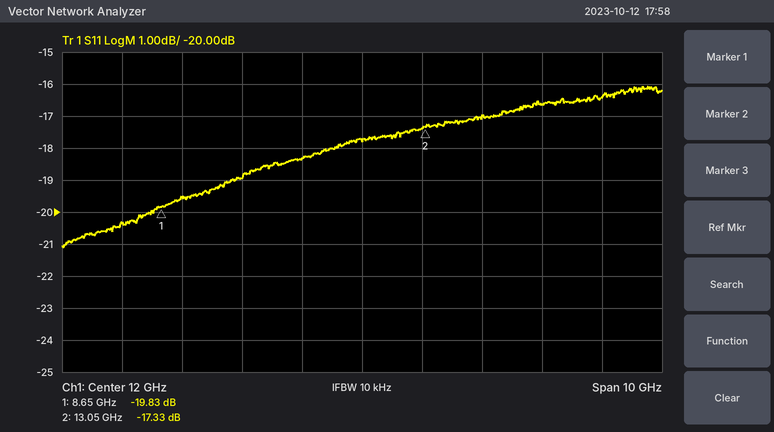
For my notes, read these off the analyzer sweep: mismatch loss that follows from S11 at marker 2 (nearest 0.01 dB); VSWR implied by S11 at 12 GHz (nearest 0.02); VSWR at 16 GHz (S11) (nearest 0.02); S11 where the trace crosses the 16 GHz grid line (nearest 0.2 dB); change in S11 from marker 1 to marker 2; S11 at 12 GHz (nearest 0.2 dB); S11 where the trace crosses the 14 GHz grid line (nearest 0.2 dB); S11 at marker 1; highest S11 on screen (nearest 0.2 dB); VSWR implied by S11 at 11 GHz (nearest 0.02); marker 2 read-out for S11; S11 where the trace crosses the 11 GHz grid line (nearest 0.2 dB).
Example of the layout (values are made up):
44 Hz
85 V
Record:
0.08 dB
1.30
1.36
-16.4 dB
2.50 dB
-17.8 dB
-17.0 dB
-19.83 dB
-16.0 dB
1.28
-17.33 dB
-18.4 dB
